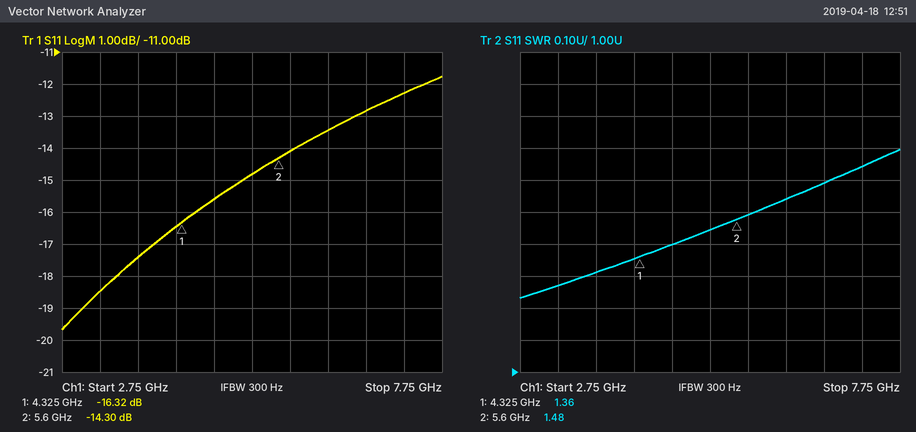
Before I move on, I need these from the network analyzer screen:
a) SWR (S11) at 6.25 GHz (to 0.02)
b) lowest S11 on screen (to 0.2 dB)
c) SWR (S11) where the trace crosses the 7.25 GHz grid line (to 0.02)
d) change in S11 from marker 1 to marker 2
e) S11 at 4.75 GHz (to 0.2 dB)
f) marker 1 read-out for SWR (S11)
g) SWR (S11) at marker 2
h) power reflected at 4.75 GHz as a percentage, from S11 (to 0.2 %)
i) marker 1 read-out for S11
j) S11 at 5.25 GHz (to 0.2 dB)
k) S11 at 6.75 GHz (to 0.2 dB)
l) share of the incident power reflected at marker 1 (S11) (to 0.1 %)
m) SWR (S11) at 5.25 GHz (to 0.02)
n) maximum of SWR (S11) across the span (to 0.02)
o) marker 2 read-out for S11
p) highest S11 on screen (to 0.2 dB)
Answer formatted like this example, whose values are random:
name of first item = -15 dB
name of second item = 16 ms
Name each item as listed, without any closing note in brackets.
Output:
SWR (S11) at 6.25 GHz = 1.54
lowest S11 on screen = -19.6 dB
SWR (S11) where the trace crosses the 7.25 GHz grid line = 1.64
change in S11 from marker 1 to marker 2 = 2.02 dB
S11 at 4.75 GHz = -15.6 dB
marker 1 read-out for SWR = 1.36
SWR (S11) at marker 2 = 1.48
power reflected at 4.75 GHz as a percentage, from S11 = 2.8 %
marker 1 read-out for S11 = -16.32 dB
S11 at 5.25 GHz = -14.8 dB
S11 at 6.75 GHz = -12.8 dB
share of the incident power reflected at marker 1 (S11) = 2.3 %
SWR (S11) at 5.25 GHz = 1.44
maximum of SWR (S11) across the span = 1.70
marker 2 read-out for S11 = -14.30 dB
highest S11 on screen = -11.8 dB
